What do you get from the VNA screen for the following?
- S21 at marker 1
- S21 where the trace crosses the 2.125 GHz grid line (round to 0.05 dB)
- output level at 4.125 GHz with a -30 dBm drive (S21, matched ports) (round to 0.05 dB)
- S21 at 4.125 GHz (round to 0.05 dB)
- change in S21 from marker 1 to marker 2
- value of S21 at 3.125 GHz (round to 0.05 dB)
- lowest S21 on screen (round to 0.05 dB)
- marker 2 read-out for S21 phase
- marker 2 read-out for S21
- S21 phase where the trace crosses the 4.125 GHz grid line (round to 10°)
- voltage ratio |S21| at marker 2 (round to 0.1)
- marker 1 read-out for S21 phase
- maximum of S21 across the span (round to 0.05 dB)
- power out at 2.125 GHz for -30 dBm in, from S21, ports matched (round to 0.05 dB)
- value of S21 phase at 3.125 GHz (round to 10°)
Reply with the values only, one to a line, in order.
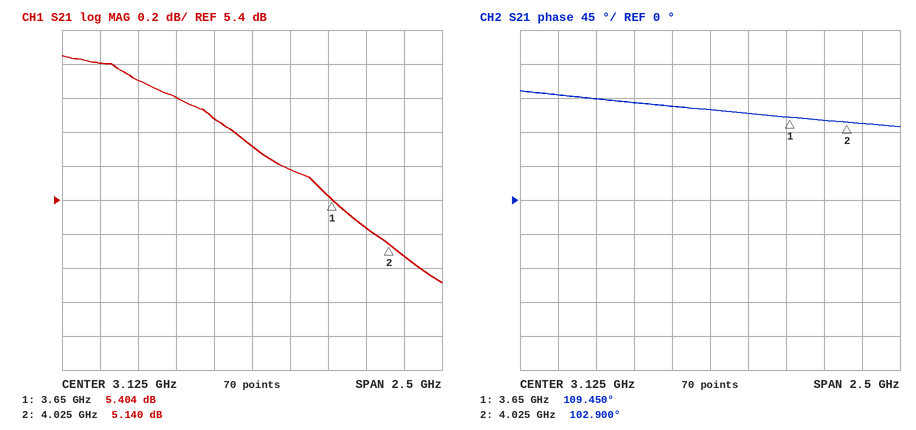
5.404 dB
6.20 dB
-24.95 dBm
5.05 dB
-0.264 dB
5.70 dB
4.90 dB
102.900°
5.140 dB
100°
1.8
109.450°
6.25 dB
-23.80 dBm
120°
